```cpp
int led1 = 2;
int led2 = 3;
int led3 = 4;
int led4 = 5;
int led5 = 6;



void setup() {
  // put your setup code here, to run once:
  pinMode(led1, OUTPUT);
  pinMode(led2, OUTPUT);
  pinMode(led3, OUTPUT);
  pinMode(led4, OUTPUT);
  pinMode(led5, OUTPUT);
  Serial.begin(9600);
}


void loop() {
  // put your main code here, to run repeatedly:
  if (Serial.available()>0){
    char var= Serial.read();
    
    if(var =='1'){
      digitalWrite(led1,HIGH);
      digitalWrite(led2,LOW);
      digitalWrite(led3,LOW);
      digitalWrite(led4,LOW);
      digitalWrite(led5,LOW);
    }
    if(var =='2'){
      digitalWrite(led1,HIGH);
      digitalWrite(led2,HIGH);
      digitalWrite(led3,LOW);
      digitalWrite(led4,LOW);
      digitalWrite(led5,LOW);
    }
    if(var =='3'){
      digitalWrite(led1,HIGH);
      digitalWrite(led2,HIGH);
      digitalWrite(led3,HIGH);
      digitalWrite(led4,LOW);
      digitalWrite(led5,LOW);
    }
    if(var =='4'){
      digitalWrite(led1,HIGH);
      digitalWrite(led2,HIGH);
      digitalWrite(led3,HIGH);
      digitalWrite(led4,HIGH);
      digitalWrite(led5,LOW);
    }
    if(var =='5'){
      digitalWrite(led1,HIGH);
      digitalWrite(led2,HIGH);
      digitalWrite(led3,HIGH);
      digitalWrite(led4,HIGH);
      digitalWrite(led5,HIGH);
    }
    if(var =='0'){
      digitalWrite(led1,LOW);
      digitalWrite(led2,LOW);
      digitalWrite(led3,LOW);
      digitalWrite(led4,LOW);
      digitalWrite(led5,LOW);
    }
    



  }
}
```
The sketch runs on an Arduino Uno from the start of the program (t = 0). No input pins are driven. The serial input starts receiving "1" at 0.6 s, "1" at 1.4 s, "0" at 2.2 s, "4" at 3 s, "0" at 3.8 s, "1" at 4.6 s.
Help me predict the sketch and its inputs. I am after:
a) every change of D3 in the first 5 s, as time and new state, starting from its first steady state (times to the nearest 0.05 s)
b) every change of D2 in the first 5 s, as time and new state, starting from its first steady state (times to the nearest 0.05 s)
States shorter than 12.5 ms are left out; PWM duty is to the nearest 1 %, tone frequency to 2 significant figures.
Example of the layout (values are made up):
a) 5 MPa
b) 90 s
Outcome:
a) 0 s low; 3 s high; 3.8 s low
b) 0 s low; 0.6 s high; 2.2 s low; 3 s high; 3.8 s low; 4.6 s high
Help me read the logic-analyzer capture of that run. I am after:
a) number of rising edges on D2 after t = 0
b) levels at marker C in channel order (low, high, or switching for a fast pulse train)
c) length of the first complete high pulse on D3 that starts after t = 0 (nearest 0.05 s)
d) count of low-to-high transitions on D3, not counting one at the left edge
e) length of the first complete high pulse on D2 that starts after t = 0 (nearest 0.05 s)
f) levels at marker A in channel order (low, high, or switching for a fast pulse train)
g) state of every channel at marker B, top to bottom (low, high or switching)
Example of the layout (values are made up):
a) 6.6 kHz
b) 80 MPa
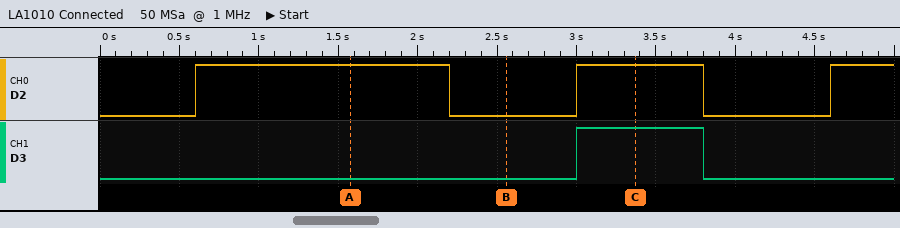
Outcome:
a) 3
b) D2 high, D3 high
c) 0.80 s
d) 1
e) 1.60 s
f) D2 high, D3 low
g) D2 low, D3 low
